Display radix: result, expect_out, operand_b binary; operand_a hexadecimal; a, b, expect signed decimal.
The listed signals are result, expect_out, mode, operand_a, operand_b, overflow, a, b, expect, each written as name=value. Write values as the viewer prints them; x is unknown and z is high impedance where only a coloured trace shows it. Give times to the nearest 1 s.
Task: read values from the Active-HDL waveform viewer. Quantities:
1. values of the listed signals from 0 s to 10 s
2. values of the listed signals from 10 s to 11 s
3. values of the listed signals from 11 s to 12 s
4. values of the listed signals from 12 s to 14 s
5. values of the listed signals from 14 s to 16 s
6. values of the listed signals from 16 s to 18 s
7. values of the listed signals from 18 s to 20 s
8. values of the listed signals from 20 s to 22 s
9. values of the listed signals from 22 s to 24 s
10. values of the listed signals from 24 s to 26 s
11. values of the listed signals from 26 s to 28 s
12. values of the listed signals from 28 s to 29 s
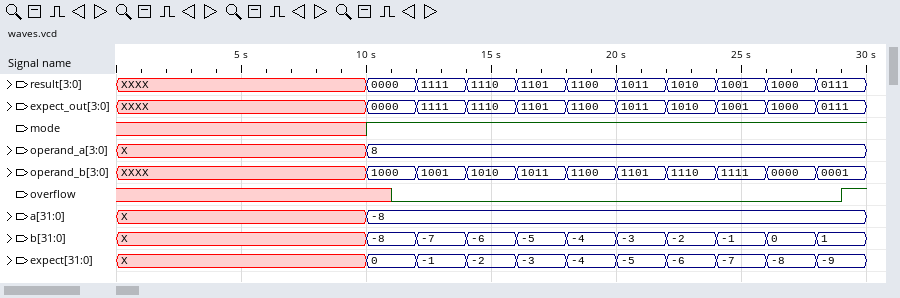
result=XXXX, expect_out=XXXX, mode=x, operand_a=X, operand_b=XXXX, overflow=x, a=X, b=X, expect=X
result=0000, expect_out=0000, mode=1, operand_a=8, operand_b=1000, overflow=x, a=-8, b=-8, expect=0
result=0000, expect_out=0000, mode=1, operand_a=8, operand_b=1000, overflow=0, a=-8, b=-8, expect=0
result=1111, expect_out=1111, mode=1, operand_a=8, operand_b=1001, overflow=0, a=-8, b=-7, expect=-1
result=1110, expect_out=1110, mode=1, operand_a=8, operand_b=1010, overflow=0, a=-8, b=-6, expect=-2
result=1101, expect_out=1101, mode=1, operand_a=8, operand_b=1011, overflow=0, a=-8, b=-5, expect=-3
result=1100, expect_out=1100, mode=1, operand_a=8, operand_b=1100, overflow=0, a=-8, b=-4, expect=-4
result=1011, expect_out=1011, mode=1, operand_a=8, operand_b=1101, overflow=0, a=-8, b=-3, expect=-5
result=1010, expect_out=1010, mode=1, operand_a=8, operand_b=1110, overflow=0, a=-8, b=-2, expect=-6
result=1001, expect_out=1001, mode=1, operand_a=8, operand_b=1111, overflow=0, a=-8, b=-1, expect=-7
result=1000, expect_out=1000, mode=1, operand_a=8, operand_b=0000, overflow=0, a=-8, b=0, expect=-8
result=0111, expect_out=0111, mode=1, operand_a=8, operand_b=0001, overflow=0, a=-8, b=1, expect=-9
